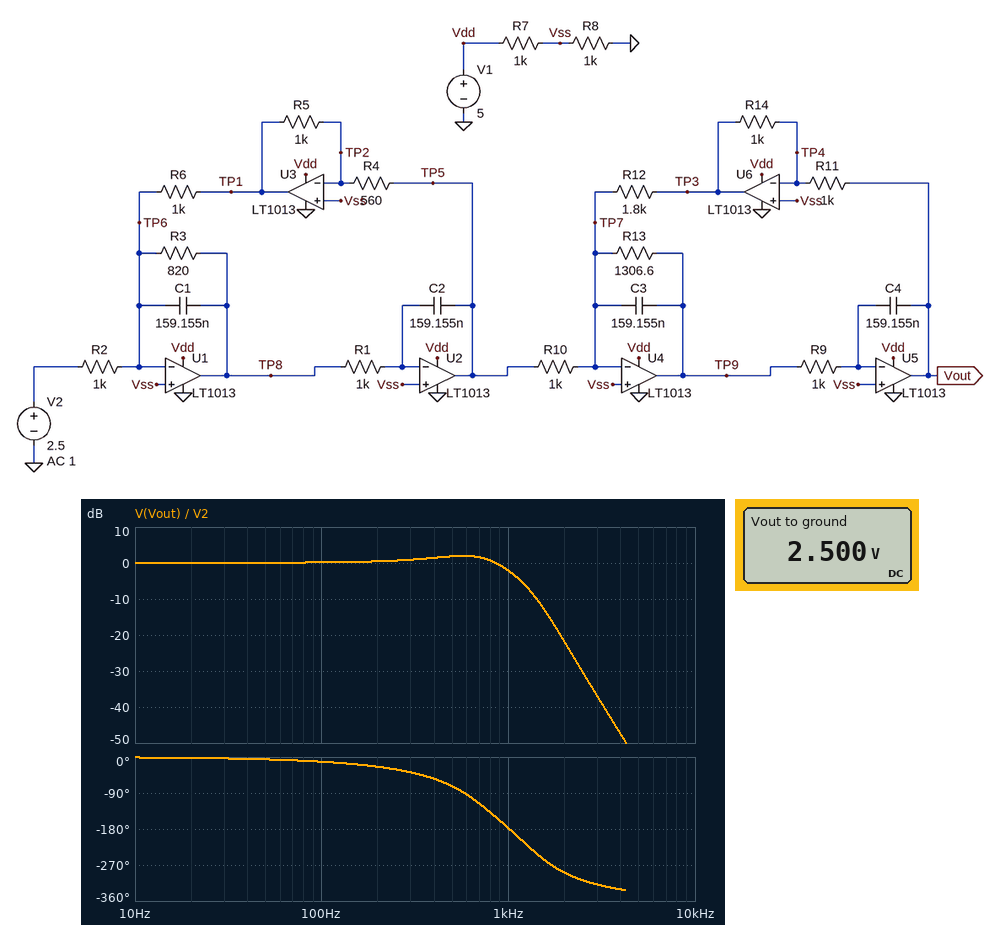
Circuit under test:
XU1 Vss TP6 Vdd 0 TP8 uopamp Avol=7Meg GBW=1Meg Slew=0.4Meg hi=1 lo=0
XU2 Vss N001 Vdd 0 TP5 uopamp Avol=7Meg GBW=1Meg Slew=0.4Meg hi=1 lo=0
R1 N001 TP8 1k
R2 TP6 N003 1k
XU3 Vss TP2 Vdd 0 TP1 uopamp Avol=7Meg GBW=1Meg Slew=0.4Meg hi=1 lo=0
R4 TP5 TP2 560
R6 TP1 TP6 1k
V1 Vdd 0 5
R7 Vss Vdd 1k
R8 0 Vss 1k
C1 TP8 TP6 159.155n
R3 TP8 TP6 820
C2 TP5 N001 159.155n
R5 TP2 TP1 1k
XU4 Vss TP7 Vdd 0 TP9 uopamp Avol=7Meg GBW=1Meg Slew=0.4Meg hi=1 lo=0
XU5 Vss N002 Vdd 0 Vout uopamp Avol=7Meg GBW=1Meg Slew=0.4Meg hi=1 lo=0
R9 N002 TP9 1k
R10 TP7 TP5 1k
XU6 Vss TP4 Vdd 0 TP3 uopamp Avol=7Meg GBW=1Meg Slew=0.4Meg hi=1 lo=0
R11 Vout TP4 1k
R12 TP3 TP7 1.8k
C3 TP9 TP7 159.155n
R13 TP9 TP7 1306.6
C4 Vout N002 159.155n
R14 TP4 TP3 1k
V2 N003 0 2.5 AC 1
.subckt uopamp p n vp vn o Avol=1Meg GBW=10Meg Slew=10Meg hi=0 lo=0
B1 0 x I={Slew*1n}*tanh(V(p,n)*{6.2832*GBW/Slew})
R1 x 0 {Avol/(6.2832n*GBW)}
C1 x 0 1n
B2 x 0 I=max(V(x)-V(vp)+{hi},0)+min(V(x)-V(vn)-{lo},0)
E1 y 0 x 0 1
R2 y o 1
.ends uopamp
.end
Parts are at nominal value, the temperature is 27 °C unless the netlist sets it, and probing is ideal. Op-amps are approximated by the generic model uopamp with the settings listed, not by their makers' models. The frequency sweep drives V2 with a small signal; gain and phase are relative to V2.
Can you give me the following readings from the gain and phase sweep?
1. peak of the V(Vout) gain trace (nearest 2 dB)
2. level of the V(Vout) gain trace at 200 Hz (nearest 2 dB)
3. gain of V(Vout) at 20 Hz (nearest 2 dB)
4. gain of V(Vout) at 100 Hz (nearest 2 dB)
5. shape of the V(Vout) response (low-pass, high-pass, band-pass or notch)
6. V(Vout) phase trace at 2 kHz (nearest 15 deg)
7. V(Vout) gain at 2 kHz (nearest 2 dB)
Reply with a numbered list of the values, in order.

1. 2 dB
2. 0 dB
3. 0 dB
4. 0 dB
5. low-pass
6. -285 deg
7. -22 dB
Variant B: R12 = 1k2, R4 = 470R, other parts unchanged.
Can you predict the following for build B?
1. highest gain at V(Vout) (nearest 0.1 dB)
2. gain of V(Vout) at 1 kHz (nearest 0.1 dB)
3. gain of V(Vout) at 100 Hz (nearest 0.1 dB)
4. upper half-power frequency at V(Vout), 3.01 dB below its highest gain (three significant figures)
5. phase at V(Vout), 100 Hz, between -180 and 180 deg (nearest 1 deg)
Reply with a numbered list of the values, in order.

1. -1.1 dB
2. -2.2 dB
3. -4.9 dB
4. 1.15 kHz
5. -9 deg
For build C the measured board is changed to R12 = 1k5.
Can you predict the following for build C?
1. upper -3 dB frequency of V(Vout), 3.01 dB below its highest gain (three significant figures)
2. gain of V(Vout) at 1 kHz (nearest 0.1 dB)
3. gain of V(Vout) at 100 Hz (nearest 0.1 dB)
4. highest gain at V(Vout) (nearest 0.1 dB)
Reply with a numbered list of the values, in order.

1. 1.01 kHz
2. -1.6 dB
3. -1.4 dB
4. 1.2 dB
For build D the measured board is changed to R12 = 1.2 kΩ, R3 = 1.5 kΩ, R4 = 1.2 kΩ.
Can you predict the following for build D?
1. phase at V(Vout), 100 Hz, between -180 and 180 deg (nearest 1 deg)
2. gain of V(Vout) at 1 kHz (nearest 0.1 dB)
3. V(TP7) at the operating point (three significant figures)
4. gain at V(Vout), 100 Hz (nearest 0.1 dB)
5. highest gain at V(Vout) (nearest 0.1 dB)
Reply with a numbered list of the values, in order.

1. -10 deg
2. 5.4 dB
3. 2.50 V
4. 3.3 dB
5. 8.9 dB
